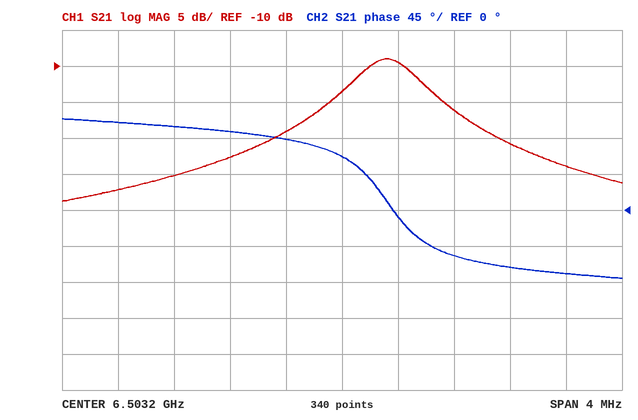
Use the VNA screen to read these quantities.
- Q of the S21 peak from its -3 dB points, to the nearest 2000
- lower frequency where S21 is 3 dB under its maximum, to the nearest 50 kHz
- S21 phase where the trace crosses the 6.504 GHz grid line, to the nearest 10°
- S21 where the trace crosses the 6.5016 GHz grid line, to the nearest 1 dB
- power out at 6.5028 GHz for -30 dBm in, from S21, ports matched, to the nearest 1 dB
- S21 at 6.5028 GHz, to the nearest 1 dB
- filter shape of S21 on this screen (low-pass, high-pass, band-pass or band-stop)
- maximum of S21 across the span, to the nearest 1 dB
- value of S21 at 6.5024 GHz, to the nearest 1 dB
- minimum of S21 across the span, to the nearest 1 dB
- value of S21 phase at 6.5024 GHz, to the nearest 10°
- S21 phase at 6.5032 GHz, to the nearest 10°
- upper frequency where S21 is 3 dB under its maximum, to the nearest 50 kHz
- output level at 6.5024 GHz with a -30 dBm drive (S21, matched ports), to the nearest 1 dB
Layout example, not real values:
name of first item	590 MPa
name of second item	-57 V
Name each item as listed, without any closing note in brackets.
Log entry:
Q of the S21 peak from its -3 dB points, to the nearest 2000	14000
lower frequency where S21 is 3 dB under its maximum, to the nearest 50 kHz	6.50330 GHz
S21 phase where the trace crosses the 6.504 GHz grid line, to the nearest 10°	-60°
S21 where the trace crosses the 6.5016 GHz grid line, to the nearest 1 dB	-27 dB
power out at 6.5028 GHz for -30 dBm in, from S21, ports matched, to the nearest 1 dB	-49 dBm
S21 at 6.5028 GHz, to the nearest 1 dB	-19 dB
filter shape of S21 on this screen	band-pass
maximum of S21 across the span, to the nearest 1 dB	-9 dB
value of S21 at 6.5024 GHz, to the nearest 1 dB	-23 dB
minimum of S21 across the span, to the nearest 1 dB	-29 dB
value of S21 phase at 6.5024 GHz, to the nearest 10°	100°
S21 phase at 6.5032 GHz, to the nearest 10°	70°
upper frequency where S21 is 3 dB under its maximum, to the nearest 50 kHz	6.50375 GHz
output level at 6.5024 GHz with a -30 dBm drive (S21, matched ports), to the nearest 1 dB	-53 dBm
